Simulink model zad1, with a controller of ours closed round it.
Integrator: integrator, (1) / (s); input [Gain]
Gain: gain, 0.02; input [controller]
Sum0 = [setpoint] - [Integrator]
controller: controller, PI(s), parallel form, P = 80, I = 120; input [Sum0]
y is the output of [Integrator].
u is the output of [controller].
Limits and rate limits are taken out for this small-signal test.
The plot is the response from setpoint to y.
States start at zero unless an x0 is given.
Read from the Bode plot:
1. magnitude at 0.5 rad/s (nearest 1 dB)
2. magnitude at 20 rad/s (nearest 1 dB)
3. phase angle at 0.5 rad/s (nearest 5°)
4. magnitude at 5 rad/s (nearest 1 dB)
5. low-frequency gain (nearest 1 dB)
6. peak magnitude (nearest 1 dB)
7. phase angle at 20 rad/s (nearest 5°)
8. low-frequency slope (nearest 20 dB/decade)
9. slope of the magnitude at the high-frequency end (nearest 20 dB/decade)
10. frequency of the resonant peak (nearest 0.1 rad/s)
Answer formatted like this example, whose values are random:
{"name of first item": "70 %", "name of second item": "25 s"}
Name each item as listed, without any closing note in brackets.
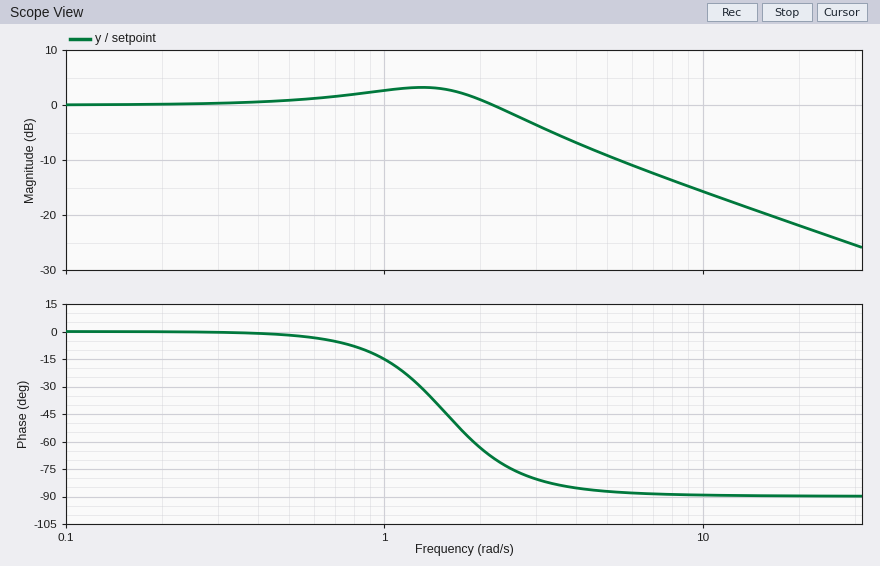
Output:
{"magnitude at 0.5 rad/s": "1 dB", "magnitude at 20 rad/s": "-22 dB", "phase angle at 0.5 rad/s": "0°", "magnitude at 5 rad/s": "-9 dB", "low-frequency gain": "0 dB", "peak magnitude": "3 dB", "phase angle at 20 rad/s": "-90°", "low-frequency slope": "0 dB/decade", "slope of the magnitude at the high-frequency end": "-20 dB/decade", "frequency of the resonant peak": "1.3 rad/s"}
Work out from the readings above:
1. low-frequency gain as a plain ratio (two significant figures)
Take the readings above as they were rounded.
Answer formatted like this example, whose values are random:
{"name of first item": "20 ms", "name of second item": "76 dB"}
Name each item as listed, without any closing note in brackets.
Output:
{"low-frequency gain as a plain ratio": "1.0"}
